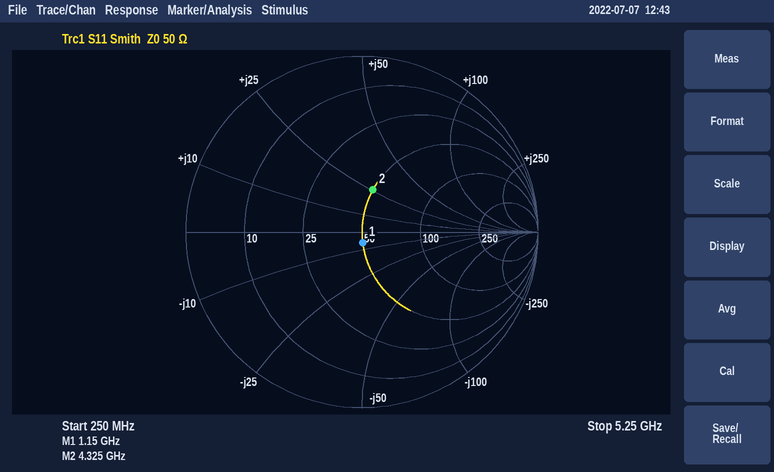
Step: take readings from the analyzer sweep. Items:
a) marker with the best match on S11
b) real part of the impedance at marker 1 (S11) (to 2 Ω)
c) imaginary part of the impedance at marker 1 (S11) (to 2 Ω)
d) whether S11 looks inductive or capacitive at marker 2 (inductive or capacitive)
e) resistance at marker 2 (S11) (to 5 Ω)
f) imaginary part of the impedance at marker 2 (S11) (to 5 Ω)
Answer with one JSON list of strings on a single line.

["marker 1", "50 Ω", "-6 Ω", "inductive", "50 Ω", "+25 Ω"]
